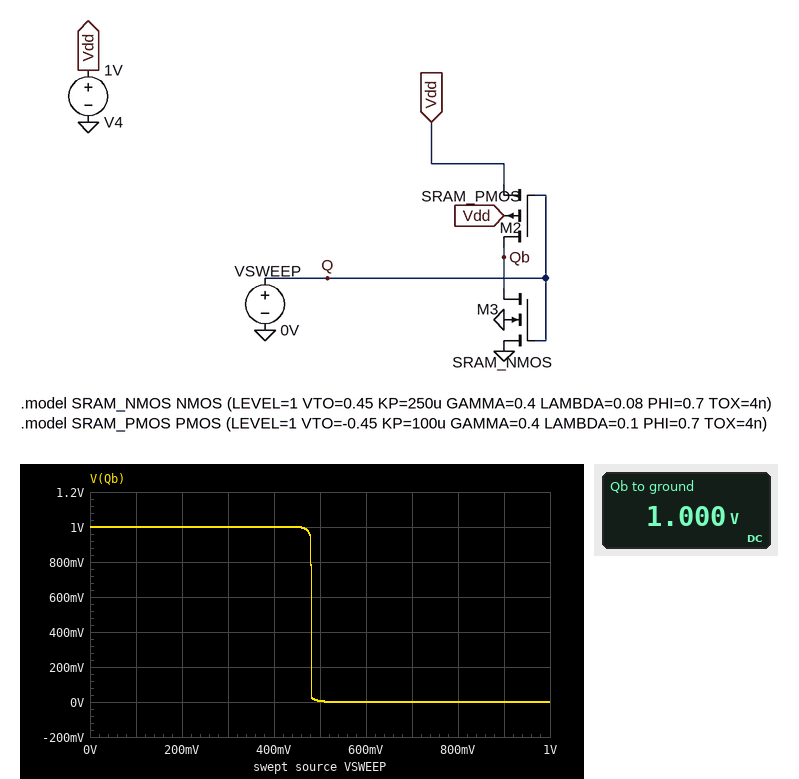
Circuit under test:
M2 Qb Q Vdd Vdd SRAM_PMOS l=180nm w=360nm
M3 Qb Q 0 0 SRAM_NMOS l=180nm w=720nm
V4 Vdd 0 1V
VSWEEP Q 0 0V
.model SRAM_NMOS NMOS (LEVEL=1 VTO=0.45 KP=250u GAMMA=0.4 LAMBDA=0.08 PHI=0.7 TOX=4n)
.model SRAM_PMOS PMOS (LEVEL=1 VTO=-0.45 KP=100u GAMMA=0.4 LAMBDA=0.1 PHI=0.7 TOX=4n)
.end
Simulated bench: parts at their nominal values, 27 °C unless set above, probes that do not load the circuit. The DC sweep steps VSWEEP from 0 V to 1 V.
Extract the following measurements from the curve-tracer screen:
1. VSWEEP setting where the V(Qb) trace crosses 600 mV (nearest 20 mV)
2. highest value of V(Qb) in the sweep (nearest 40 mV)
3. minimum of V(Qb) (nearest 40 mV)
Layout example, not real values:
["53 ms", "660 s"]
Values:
["480 mV", "1.00 V", "0 V"]
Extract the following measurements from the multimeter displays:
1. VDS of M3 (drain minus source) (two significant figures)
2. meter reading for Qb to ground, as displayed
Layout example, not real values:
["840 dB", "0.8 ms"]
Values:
["1.0 V", "1.000 V"]
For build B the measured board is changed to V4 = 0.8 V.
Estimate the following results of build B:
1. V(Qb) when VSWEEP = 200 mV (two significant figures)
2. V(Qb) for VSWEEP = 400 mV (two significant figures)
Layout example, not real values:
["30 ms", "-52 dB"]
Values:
["800 mV", "400 mV"]
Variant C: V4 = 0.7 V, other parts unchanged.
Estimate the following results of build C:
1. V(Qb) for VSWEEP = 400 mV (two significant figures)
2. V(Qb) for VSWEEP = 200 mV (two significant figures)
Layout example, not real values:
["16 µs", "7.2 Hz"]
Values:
["350 mV", "700 mV"]
